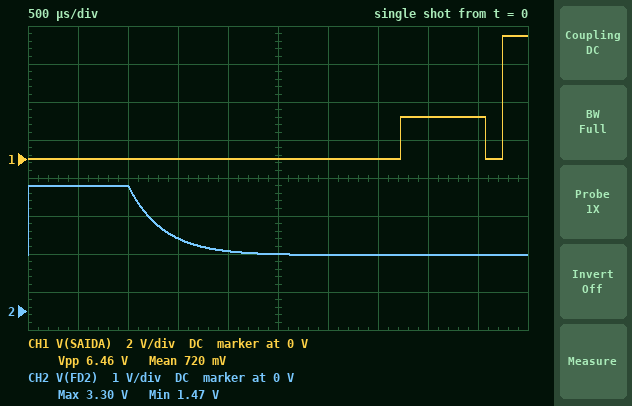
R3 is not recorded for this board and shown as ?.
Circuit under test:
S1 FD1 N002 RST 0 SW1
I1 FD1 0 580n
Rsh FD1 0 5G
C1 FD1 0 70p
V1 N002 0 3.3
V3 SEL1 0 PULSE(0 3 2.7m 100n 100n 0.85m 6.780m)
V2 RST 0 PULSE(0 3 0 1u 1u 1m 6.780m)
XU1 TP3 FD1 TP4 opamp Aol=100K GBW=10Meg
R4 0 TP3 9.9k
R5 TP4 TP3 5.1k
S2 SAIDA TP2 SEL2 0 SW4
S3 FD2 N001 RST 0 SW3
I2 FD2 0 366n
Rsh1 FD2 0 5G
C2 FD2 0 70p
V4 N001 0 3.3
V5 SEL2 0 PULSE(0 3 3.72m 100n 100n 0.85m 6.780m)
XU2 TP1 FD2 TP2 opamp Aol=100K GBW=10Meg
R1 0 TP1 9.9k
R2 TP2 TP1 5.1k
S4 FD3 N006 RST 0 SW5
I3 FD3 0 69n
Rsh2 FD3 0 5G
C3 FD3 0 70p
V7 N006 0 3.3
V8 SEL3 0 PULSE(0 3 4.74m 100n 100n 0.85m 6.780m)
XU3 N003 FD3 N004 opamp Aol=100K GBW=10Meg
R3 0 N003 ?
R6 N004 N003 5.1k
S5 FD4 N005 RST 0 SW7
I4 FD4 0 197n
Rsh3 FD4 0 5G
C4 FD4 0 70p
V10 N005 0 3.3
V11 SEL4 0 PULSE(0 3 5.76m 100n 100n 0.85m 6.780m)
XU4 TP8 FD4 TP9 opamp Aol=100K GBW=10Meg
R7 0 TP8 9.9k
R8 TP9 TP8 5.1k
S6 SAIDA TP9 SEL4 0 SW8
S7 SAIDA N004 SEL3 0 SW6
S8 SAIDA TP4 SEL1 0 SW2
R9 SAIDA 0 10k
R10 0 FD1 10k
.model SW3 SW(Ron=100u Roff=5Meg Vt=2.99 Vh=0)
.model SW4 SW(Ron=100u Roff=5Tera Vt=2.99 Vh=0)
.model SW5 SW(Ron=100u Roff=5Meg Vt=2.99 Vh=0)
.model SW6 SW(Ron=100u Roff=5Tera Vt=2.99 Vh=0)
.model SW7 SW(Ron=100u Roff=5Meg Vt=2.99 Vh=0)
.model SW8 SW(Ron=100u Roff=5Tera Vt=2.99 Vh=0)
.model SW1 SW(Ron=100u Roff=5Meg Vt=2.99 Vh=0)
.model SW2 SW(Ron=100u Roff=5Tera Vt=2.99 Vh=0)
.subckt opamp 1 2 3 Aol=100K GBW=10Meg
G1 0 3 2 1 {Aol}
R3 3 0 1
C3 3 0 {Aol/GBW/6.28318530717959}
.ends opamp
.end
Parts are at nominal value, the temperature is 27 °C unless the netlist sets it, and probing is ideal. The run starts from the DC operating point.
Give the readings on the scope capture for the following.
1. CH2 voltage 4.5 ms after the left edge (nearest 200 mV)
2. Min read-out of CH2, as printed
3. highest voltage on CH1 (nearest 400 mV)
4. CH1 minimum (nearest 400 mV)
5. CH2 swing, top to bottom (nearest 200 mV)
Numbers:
1.4 V
1.47 V
6.4 V
0 V
1.8 V
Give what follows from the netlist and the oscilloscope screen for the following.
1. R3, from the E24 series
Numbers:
4.3 kΩ
